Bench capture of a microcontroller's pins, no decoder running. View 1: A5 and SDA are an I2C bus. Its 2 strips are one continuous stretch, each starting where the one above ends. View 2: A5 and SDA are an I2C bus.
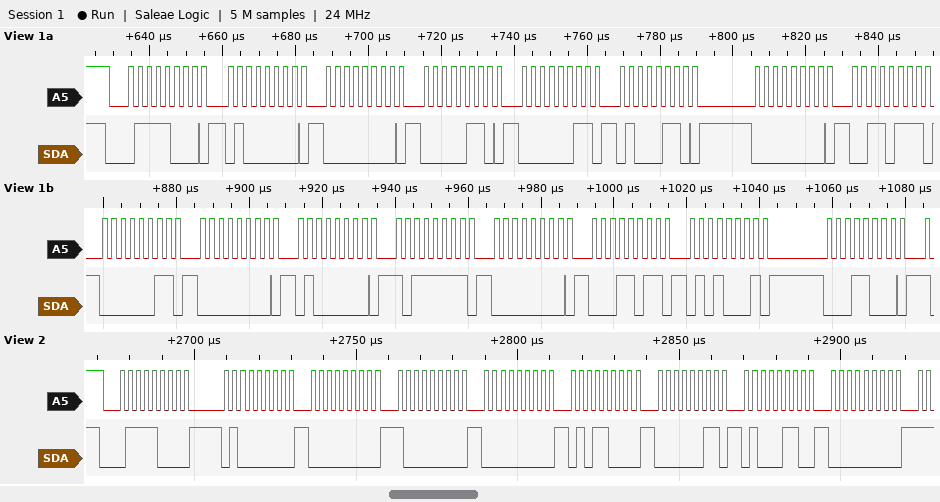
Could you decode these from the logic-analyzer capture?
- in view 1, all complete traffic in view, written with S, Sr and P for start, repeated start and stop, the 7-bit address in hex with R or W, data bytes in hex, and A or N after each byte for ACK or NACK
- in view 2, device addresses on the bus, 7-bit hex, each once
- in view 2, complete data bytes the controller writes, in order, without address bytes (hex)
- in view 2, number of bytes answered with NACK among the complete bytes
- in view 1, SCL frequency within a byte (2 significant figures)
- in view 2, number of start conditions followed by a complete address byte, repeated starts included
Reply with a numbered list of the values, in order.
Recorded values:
1. S 3CW A 40 A 00 A 06 A 03 A 46 A 00 A 37 A 03 A 00 A 40 A BF A 00 A 1B A 51 A 18 A
2. 0x3C
3. 40 00 80 00 58 03 46 00
4. 0
5. 400 kHz
6. 1
